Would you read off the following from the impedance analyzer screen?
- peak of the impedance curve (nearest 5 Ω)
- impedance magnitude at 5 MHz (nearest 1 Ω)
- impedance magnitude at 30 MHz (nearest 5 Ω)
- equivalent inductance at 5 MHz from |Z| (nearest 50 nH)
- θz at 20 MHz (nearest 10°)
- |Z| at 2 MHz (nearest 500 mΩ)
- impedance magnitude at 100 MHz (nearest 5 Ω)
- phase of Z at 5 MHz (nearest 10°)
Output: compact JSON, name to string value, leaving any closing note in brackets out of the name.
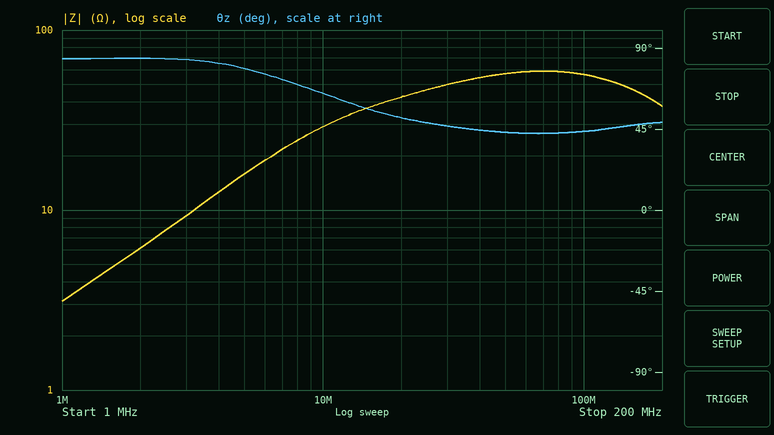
{"peak of the impedance curve": "60 Ω", "impedance magnitude at 5 MHz": "16 Ω", "impedance magnitude at 30 MHz": "50 Ω", "equivalent inductance at 5 MHz from |Z|": "500 nH", "θz at 20 MHz": "50°", "|Z| at 2 MHz": "6.0 Ω", "impedance magnitude at 100 MHz": "55 Ω", "phase of Z at 5 MHz": "80°"}
